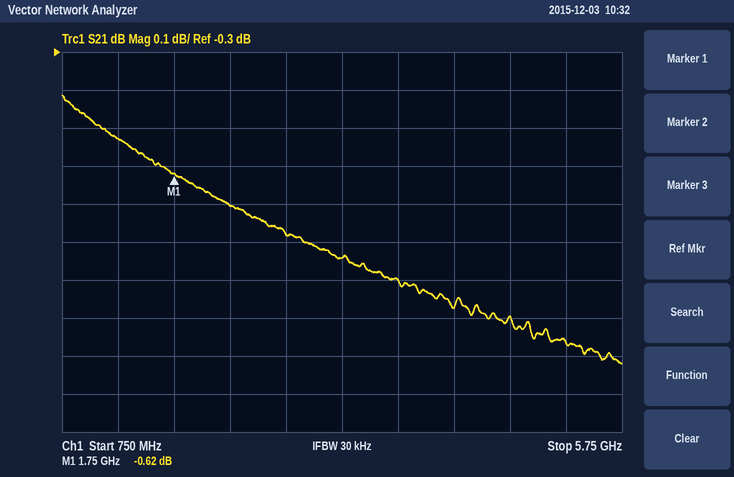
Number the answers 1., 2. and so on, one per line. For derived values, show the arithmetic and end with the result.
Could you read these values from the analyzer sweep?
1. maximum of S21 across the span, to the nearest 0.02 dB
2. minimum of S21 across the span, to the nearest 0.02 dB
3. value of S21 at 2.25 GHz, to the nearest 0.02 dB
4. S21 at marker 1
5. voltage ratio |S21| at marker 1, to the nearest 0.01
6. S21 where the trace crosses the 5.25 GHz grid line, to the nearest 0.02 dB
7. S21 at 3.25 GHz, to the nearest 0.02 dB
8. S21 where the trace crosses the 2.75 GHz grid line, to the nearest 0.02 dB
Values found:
1. -0.42 dB
2. -1.12 dB
3. -0.70 dB
4. -0.62 dB
5. 10^(-0.62/20) ≈ 0.93
6. -1.06 dB
7. -0.84 dB
8. -0.78 dB
